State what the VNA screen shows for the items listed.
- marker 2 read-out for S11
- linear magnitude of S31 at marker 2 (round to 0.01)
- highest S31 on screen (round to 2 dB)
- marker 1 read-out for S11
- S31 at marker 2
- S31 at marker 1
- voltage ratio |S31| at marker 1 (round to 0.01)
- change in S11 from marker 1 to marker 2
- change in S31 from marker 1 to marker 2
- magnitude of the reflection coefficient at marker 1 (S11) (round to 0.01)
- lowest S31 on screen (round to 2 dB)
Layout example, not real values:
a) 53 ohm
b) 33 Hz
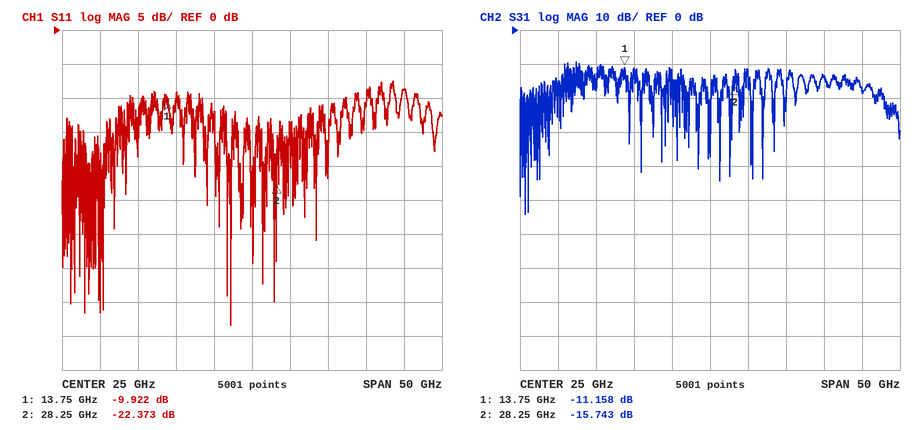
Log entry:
a) -22.373 dB
b) 0.16
c) -10 dB
d) -9.922 dB
e) -15.743 dB
f) -11.158 dB
g) 0.28
h) -12.451 dB
i) -4.585 dB
j) 0.32
k) -54 dB
